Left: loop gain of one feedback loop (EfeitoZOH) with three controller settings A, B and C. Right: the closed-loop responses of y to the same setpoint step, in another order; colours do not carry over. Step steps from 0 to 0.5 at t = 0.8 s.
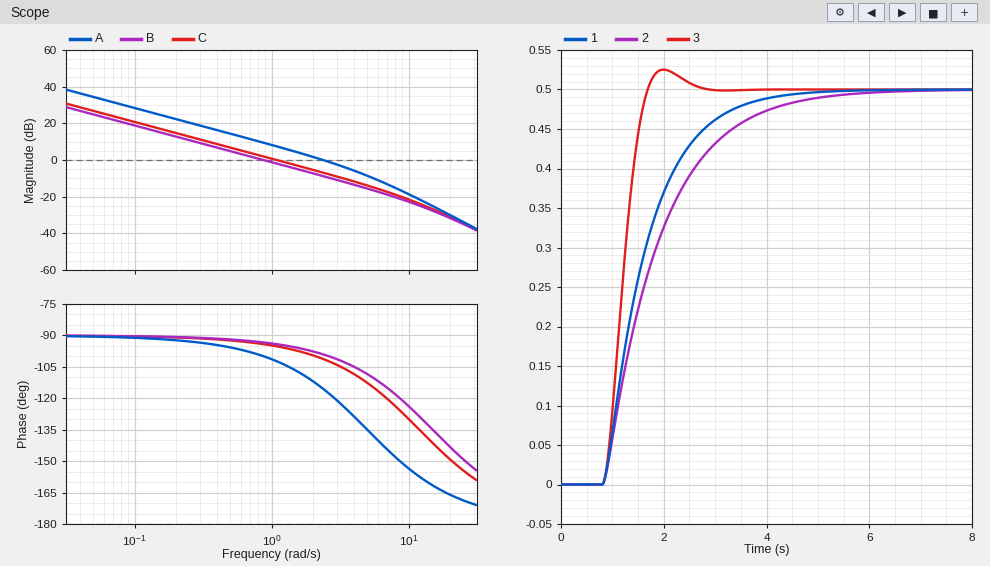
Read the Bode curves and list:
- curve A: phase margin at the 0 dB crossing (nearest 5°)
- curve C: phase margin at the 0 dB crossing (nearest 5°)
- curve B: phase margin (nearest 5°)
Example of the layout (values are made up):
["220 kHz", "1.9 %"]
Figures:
["65°", "85°", "85°"]
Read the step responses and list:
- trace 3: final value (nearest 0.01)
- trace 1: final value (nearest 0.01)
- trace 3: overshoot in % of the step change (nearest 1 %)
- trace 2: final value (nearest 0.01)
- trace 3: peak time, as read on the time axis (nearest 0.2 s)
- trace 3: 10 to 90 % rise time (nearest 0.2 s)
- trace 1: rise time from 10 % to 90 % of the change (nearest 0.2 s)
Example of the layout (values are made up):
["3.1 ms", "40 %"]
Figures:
["0.50", "0.50", "5 %", "0.50", "2.0 s", "0.6 s", "1.8 s"]
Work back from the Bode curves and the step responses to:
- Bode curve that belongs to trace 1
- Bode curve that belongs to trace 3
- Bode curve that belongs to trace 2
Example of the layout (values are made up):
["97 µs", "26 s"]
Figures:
["C", "A", "B"]
